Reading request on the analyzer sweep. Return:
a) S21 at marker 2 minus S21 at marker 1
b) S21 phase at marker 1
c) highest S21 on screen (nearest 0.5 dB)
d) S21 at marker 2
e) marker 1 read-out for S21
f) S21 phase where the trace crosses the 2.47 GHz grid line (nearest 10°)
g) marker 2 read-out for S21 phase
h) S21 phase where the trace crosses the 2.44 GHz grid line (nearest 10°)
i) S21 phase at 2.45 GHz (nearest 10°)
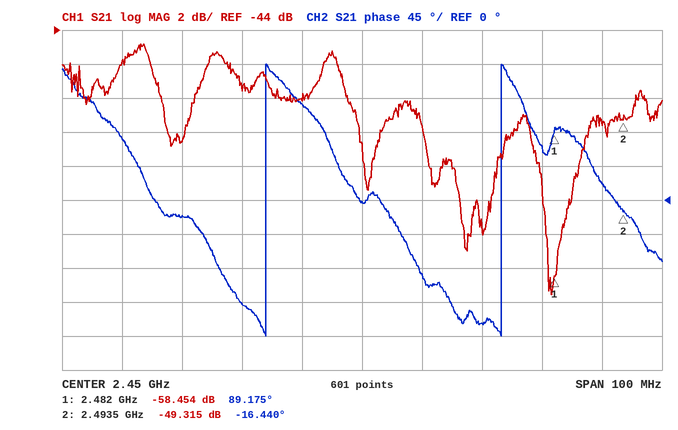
9.139 dB
89.175°
-45.0 dB
-49.315 dB
-58.454 dB
-160°
-16.440°
130°
0°
